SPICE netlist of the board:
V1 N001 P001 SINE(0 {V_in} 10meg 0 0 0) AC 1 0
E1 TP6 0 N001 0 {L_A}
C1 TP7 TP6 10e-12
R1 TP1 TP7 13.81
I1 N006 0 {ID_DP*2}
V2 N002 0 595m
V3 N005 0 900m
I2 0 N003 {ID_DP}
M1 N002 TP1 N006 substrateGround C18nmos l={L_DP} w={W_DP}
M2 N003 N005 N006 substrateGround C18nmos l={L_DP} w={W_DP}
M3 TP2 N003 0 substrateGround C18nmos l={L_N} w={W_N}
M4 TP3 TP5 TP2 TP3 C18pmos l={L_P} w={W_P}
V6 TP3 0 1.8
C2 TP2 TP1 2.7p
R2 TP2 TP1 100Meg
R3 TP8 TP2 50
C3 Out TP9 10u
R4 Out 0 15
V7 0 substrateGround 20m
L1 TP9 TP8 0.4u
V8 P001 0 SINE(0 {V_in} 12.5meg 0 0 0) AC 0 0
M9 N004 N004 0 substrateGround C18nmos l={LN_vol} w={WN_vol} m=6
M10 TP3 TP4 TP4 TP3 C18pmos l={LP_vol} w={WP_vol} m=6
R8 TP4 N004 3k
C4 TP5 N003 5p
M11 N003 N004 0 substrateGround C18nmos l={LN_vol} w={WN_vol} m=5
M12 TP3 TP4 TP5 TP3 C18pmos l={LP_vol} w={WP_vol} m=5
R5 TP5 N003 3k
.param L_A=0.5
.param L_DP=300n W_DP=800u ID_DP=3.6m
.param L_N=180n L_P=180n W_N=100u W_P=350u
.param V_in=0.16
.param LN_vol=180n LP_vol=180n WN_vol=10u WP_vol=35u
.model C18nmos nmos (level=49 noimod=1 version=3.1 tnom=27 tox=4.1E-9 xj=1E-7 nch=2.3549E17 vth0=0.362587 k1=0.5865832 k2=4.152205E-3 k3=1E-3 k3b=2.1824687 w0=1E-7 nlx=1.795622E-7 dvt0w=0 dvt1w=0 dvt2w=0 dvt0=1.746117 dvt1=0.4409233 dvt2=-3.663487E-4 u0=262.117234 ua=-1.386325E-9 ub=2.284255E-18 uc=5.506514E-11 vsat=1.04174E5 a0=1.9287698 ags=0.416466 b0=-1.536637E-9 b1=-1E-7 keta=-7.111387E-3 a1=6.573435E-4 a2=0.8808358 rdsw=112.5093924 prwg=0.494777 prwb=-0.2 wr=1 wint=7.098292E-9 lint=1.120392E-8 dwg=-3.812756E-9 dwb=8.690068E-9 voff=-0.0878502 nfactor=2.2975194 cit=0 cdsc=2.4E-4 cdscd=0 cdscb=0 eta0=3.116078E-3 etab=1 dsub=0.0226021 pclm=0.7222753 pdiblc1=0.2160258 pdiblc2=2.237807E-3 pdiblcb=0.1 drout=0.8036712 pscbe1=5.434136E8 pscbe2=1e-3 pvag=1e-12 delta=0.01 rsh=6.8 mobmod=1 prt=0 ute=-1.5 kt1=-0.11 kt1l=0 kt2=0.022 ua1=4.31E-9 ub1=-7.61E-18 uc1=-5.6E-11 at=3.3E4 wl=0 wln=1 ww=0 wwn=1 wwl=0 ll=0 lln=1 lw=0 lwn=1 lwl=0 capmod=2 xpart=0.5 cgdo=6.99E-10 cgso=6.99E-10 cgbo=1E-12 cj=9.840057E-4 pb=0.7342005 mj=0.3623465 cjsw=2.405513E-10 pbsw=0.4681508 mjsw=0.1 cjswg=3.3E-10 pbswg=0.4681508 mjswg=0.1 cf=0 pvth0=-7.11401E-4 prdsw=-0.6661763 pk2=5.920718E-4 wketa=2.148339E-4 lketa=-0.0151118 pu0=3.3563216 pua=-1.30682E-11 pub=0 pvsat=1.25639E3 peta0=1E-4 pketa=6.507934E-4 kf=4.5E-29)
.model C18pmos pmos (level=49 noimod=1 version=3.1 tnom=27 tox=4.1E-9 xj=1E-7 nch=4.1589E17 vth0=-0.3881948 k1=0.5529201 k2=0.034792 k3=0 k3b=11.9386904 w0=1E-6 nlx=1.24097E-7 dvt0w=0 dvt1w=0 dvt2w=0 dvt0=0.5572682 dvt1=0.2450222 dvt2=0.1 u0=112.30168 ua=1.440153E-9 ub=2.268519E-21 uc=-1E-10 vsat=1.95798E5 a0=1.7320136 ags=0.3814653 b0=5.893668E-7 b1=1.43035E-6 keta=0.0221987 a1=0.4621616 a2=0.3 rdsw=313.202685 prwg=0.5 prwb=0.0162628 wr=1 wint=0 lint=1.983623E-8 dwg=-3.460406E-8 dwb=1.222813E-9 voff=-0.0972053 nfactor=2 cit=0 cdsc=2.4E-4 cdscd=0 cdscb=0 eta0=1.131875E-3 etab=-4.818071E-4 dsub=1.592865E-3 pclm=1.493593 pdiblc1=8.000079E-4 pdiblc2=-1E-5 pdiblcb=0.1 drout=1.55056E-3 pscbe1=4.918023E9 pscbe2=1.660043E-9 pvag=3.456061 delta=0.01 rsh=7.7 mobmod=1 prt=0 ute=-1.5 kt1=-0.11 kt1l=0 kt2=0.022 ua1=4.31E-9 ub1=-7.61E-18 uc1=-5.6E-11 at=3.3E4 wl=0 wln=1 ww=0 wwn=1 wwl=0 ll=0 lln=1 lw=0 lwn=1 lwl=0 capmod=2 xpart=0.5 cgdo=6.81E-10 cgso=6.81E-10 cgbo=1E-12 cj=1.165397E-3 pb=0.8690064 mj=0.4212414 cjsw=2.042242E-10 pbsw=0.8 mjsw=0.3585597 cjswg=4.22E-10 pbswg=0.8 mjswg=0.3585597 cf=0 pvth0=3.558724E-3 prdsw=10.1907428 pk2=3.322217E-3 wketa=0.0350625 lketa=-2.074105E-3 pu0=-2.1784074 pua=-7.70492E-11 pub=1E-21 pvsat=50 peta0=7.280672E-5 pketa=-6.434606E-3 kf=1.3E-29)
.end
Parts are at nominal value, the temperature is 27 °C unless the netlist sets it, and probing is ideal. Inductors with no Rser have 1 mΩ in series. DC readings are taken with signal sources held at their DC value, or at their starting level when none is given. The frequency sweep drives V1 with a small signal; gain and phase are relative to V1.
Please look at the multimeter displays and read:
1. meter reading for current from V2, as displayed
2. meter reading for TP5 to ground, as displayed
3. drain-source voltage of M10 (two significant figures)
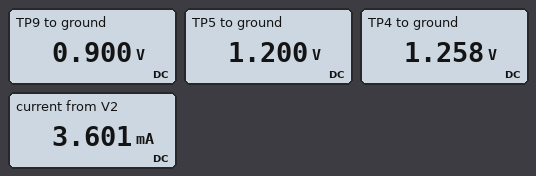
3.601 mA
1.200 V
540 mV
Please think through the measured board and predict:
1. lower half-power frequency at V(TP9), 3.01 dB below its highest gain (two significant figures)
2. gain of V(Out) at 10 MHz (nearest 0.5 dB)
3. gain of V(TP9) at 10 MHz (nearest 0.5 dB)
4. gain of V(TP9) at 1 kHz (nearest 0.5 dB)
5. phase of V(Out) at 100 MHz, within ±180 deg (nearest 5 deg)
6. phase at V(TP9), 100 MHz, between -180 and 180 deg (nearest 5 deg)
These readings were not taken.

160 Hz
-8.5 dB
-8.5 dB
-6.0 dB
95 deg
95 deg
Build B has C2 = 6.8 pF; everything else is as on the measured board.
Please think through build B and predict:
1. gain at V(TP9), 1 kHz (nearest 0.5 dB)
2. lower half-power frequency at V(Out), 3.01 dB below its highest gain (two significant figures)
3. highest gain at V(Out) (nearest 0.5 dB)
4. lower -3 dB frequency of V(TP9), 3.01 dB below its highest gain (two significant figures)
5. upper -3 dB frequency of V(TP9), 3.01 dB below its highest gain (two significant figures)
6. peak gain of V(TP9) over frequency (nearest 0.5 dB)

-13.0 dB
360 Hz
-15.5 dB
100 Hz
690 Hz
-8.5 dB
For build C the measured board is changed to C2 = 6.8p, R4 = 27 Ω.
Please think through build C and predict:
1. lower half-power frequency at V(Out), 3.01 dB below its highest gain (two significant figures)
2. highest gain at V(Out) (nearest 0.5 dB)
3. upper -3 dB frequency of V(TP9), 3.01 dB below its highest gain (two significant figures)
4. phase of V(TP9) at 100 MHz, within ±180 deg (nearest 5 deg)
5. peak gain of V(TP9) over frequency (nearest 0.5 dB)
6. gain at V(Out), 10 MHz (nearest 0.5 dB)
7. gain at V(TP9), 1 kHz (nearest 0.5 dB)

340 Hz
-12.0 dB
1.8 kHz
100 deg
-8.5 dB
-12.5 dB
-11.0 dB
